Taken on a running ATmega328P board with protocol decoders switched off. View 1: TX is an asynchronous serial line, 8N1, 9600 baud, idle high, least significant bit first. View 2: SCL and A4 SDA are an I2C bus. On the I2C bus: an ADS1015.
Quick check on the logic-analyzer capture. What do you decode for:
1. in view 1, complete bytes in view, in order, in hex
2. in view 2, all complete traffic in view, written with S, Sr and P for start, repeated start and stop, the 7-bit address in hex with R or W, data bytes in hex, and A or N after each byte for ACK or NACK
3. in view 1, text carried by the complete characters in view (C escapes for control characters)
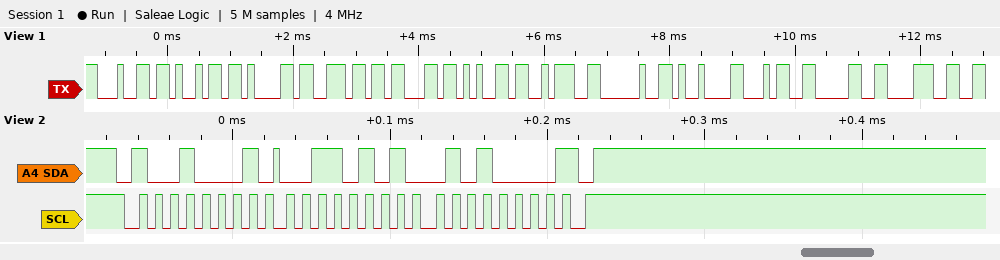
64 69 61 6E 63 65 3A 20 09 34 30 38
S 48R A 35 A 50 N P
"diance: \t408"
